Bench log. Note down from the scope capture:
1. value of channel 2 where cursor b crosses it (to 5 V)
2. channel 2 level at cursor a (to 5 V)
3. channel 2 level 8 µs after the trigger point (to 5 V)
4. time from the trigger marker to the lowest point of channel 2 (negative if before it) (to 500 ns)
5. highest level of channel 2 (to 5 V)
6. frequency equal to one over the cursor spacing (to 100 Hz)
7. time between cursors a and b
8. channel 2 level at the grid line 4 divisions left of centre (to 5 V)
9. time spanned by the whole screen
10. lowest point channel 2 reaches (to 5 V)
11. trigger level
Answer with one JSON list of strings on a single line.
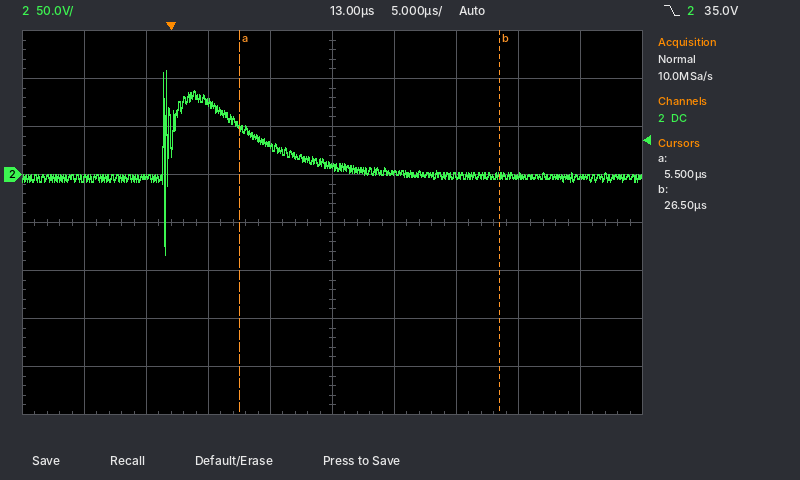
["0 V", "50 V", "30 V", "-500 ns", "110 V", "47.6 kHz", "21.0 µs", "-5 V", "50 µs", "-85 V", "35.0 V"]
